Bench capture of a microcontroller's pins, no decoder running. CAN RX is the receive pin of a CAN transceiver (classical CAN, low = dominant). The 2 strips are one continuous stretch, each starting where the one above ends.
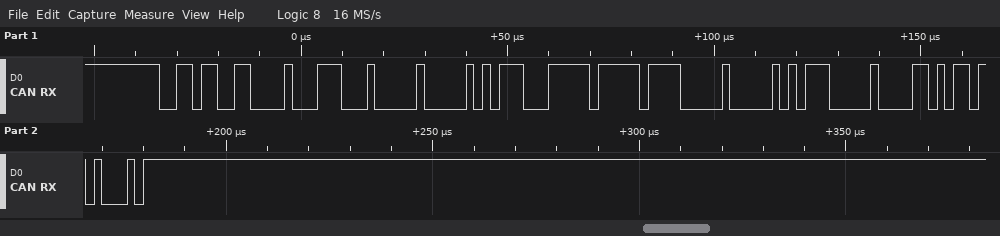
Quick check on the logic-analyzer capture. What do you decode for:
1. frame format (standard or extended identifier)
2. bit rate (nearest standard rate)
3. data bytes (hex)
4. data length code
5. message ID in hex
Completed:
standard
500 kbit/s
E2 00 2E 3F FF 00 17 00
8
0x366
